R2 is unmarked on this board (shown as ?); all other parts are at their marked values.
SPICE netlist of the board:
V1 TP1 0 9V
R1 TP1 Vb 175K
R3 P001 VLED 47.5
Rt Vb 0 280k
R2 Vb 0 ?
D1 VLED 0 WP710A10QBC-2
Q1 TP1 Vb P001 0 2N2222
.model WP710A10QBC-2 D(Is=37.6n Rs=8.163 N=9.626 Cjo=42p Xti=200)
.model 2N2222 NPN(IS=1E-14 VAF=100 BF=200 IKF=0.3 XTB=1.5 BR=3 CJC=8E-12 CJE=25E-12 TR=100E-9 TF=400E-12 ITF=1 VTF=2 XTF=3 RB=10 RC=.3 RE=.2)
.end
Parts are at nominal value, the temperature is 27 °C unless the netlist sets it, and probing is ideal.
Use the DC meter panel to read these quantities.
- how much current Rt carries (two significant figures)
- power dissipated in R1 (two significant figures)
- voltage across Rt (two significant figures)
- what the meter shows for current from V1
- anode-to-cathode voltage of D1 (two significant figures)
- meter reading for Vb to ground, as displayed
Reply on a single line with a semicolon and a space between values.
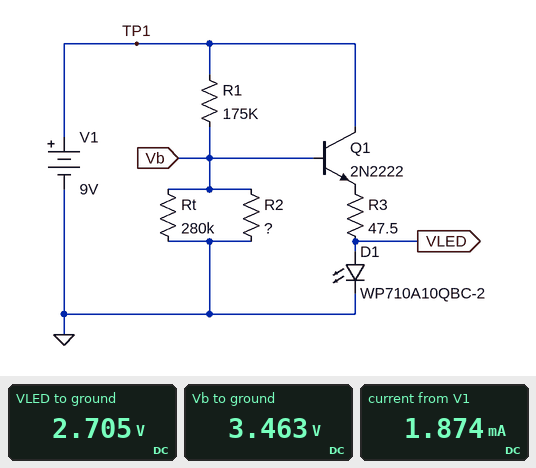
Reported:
12 µA; 180 µW; 3.5 V; 1.874 mA; 2.7 V; 3.463 V
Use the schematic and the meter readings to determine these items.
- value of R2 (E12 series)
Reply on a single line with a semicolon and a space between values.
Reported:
330 kΩ
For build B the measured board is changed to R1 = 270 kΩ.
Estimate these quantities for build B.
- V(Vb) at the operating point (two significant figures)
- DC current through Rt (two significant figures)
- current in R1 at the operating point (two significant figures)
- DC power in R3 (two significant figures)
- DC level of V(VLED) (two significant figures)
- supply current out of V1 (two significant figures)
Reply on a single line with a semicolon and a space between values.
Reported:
3.0 V; 11 µA; 22 µA; 11 µW; 2.4 V; 500 µA
